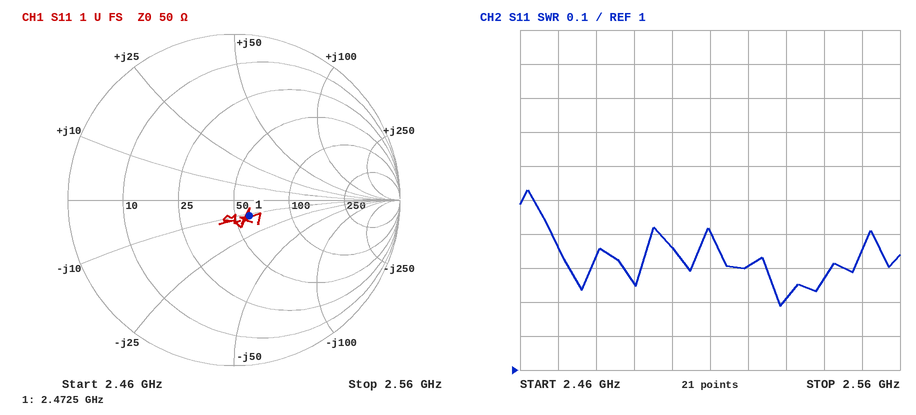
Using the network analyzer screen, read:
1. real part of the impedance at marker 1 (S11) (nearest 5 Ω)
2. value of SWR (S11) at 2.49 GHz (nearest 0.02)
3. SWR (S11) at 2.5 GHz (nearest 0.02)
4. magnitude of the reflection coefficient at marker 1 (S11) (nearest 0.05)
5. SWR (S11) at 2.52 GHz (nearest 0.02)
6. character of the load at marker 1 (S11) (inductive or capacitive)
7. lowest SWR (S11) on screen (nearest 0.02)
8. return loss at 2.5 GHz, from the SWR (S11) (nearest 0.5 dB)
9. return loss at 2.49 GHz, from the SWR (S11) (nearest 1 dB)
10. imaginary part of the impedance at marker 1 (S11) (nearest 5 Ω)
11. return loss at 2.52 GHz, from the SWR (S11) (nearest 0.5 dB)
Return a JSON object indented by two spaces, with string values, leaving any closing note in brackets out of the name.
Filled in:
{
  "real part of the impedance at marker 1 (S11)": "60 Ω",
  "value of SWR (S11) at 2.49 GHz": "1.26",
  "SWR (S11) at 2.5 GHz": "1.36",
  "magnitude of the reflection coefficient at marker 1 (S11)": "0.15",
  "SWR (S11) at 2.52 GHz": "1.30",
  "character of the load at marker 1 (S11)": "capacitive",
  "lowest SWR (S11) on screen": "1.18",
  "return loss at 2.5 GHz, from the SWR (S11)": "16.5 dB",
  "return loss at 2.49 GHz, from the SWR (S11)": "19 dB",
  "imaginary part of the impedance at marker 1 (S11)": "-10 Ω",
  "return loss at 2.52 GHz, from the SWR (S11)": "17.5 dB"
}
